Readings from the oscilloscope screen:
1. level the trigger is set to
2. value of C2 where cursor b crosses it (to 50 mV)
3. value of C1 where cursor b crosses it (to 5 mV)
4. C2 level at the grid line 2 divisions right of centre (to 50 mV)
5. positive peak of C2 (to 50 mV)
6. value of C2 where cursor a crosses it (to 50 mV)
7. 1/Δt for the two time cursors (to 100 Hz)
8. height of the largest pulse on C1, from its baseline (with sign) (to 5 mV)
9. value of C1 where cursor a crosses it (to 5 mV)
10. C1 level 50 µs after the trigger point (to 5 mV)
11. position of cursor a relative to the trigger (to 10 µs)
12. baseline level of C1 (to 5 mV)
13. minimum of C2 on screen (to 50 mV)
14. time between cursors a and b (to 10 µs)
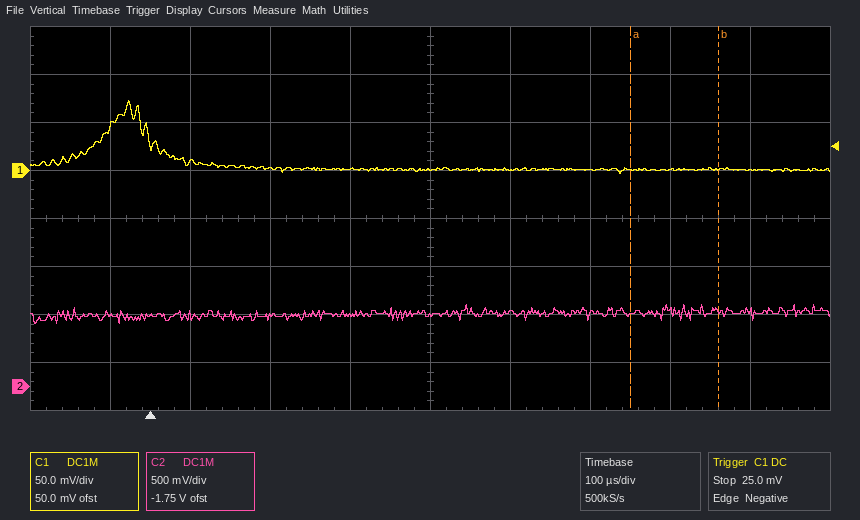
25.0 mV
800 mV
0 mV
750 mV
850 mV
750 mV
9.1 kHz
+70 mV
0 mV
10 mV
+600 µs
0 mV
650 mV
110 µs
